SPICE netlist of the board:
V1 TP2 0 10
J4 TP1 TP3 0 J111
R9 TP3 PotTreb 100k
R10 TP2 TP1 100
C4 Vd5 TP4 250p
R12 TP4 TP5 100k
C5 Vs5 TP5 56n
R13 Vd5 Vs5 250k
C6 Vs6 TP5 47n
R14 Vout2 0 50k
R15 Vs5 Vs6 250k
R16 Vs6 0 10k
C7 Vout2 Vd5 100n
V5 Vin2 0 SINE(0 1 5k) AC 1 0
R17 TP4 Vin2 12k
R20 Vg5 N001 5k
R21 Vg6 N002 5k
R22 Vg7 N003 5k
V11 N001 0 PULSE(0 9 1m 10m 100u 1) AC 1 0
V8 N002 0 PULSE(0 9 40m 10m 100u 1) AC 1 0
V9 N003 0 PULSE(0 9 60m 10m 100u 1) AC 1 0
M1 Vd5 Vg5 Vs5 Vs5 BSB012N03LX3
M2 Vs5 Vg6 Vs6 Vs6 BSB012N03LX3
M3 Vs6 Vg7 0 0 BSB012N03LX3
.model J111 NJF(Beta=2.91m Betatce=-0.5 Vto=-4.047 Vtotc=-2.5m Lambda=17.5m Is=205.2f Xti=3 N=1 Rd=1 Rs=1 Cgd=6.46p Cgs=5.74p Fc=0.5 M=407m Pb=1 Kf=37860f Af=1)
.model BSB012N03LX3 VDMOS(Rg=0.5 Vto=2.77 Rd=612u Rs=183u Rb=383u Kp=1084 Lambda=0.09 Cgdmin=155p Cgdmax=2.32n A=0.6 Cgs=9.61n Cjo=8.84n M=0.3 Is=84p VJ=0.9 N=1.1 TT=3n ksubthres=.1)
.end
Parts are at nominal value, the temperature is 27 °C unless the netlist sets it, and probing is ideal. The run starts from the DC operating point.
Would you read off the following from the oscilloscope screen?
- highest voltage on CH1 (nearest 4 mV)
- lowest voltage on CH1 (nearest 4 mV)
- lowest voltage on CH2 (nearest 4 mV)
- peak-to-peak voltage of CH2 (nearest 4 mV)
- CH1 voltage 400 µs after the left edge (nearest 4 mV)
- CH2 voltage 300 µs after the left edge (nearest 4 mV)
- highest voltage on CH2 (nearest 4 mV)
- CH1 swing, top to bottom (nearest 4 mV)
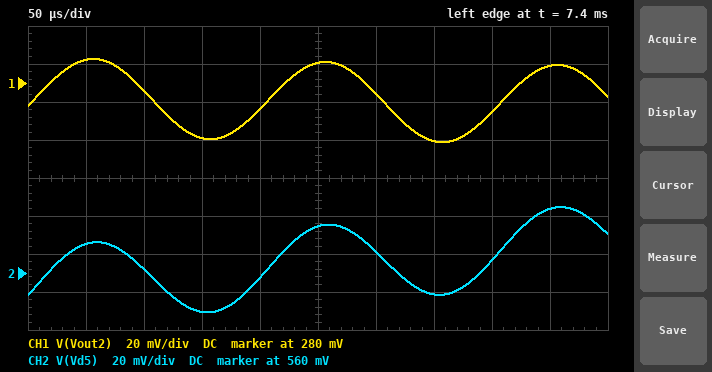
292 mV
248 mV
540 mV
56 mV
264 mV
572 mV
596 mV
44 mV
